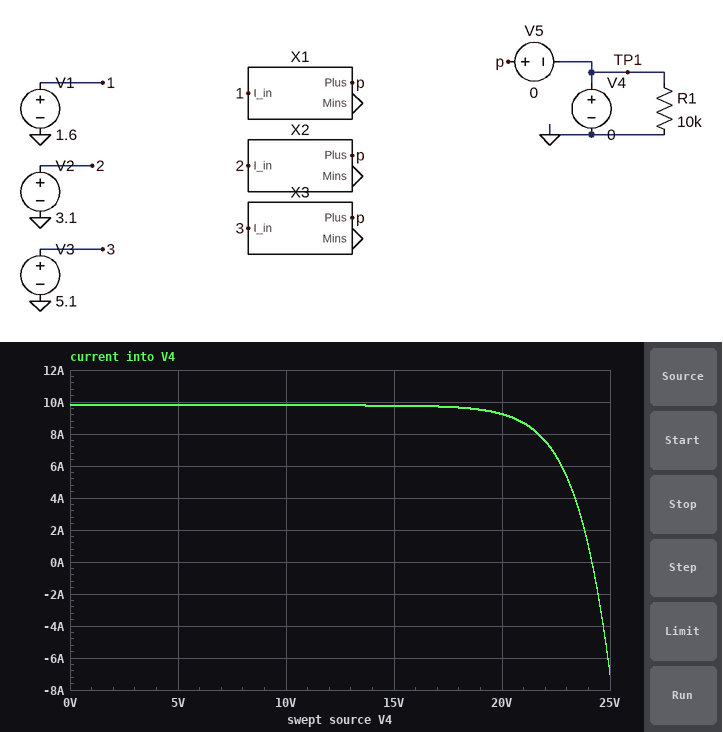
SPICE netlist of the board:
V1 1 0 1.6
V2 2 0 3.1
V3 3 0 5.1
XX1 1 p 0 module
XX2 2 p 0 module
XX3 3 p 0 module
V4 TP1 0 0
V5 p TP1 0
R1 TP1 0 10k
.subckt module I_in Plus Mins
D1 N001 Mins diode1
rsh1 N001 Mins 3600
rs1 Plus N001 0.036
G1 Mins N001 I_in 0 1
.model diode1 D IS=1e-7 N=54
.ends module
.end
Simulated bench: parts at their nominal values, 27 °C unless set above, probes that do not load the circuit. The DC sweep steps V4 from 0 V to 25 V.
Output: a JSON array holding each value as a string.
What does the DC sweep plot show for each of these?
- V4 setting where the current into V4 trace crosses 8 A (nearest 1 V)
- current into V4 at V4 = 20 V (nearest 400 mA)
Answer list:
["22 V", "9.2 A"]
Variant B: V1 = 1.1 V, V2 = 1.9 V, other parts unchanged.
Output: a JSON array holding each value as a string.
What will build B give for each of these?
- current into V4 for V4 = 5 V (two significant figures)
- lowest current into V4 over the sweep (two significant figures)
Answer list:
["8.1 A", "-8.5 A"]
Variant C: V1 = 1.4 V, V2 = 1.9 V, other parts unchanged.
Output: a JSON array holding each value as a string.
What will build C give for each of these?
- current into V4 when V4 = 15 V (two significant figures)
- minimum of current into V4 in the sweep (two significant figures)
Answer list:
["8.4 A", "-8.2 A"]
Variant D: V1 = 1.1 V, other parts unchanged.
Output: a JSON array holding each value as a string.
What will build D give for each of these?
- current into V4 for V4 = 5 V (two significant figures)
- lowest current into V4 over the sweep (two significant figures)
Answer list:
["9.3 A", "-7.4 A"]
